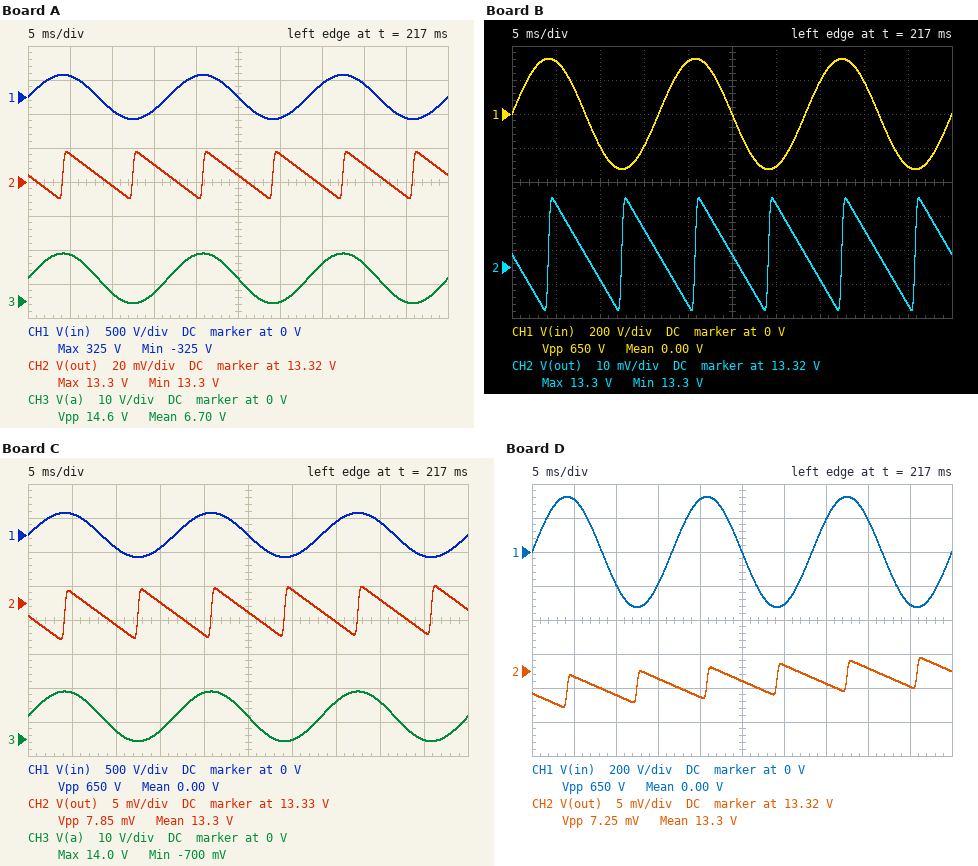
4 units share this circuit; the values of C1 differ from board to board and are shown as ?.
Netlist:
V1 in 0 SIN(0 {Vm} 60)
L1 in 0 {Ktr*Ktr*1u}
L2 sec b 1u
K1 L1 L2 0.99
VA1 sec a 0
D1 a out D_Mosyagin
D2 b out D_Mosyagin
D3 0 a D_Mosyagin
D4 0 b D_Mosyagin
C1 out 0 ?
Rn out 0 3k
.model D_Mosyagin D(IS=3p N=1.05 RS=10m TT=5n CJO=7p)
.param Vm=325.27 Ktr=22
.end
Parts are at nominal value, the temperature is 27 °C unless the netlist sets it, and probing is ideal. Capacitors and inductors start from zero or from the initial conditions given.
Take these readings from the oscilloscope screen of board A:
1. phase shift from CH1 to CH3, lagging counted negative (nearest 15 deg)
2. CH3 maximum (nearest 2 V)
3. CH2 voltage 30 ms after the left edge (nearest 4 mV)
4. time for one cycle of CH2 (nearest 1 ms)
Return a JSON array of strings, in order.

["0 deg", "14 V", "13.336 V", "8 ms"]
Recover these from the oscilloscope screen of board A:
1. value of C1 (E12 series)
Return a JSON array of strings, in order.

["1.2 mF"]
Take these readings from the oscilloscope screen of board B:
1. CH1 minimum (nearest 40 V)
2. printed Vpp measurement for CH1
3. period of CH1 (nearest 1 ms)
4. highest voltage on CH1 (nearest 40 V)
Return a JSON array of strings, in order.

["-320 V", "650 V", "17 ms", "320 V"]
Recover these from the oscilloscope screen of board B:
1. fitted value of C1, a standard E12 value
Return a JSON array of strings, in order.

["1 mF"]
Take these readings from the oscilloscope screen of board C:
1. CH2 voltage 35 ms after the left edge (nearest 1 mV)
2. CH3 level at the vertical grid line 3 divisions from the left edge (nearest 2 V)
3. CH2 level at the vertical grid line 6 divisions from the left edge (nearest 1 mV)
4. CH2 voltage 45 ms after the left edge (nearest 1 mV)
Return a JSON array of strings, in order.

["13.322 V", "2 V", "13.327 V", "13.321 V"]
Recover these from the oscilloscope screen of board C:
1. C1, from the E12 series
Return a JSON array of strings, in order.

["4.7 mF"]
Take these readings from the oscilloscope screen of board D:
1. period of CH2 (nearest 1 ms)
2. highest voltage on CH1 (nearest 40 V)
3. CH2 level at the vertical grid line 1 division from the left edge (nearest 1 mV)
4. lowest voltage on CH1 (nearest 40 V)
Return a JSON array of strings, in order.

["8 ms", "320 V", "13.319 V", "-320 V"]
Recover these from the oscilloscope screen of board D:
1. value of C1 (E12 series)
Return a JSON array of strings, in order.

["8.2 mF"]
